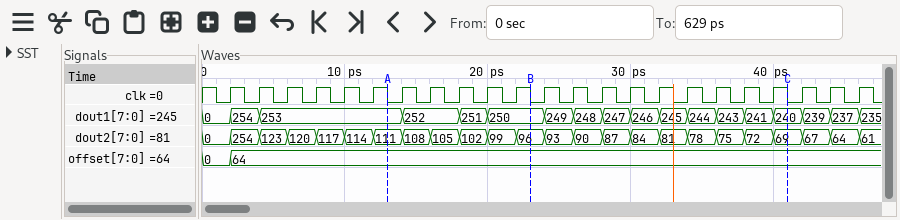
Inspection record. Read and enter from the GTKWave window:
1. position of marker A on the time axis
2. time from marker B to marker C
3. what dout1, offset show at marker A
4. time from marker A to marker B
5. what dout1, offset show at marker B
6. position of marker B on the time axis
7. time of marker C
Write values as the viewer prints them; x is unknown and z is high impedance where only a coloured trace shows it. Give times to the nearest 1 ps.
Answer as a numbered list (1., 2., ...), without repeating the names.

1. 13 ps
2. 18 ps
3. dout1=253, offset=64
4. 10 ps
5. dout1=250, offset=64
6. 23 ps
7. 41 ps
